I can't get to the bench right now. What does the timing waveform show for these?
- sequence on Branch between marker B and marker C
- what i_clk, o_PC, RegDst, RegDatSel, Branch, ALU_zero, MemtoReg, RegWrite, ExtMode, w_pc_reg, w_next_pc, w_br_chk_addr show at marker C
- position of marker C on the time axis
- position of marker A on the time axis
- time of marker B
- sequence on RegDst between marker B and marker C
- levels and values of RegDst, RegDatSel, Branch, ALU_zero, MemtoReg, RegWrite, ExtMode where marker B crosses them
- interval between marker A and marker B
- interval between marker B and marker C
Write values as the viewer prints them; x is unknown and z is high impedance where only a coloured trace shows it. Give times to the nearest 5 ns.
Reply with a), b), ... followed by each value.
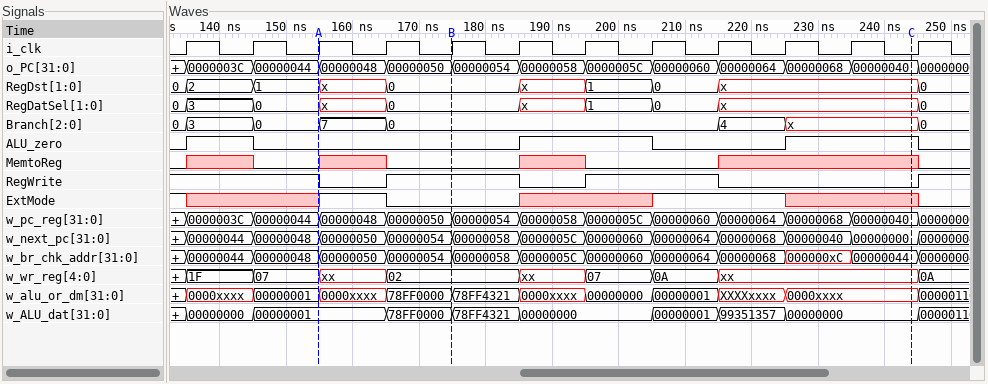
a) 0, 4, x
b) i_clk=0, o_PC=00000040, RegDst=x, RegDatSel=x, Branch=x, ALU_zero=1, MemtoReg=x, RegWrite=0, ExtMode=x, w_pc_reg=00000040, w_next_pc=00000000, w_br_chk_addr=00000044
c) 245 ns
d) 155 ns
e) 175 ns
f) 0, x, 1, 0, x
g) RegDst=0, RegDatSel=0, Branch=0, ALU_zero=0, MemtoReg=0, RegWrite=1, ExtMode=0
h) 20 ns
i) 70 ns
